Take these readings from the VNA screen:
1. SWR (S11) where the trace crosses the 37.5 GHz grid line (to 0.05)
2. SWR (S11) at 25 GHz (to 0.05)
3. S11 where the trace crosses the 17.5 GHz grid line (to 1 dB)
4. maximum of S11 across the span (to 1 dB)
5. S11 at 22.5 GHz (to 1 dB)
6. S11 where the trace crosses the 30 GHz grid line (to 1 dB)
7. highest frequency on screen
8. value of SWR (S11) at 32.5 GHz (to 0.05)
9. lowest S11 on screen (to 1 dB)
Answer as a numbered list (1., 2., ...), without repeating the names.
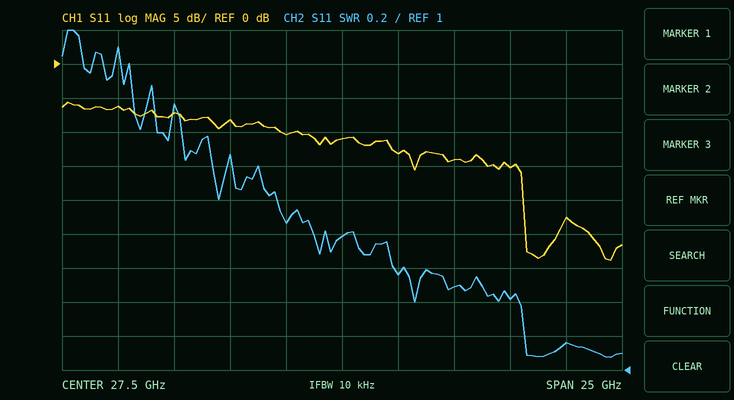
1. 1.15
2. 1.85
3. -6 dB
4. -6 dB
5. -8 dB
6. -13 dB
7. 40 GHz
8. 1.50
9. -29 dB
